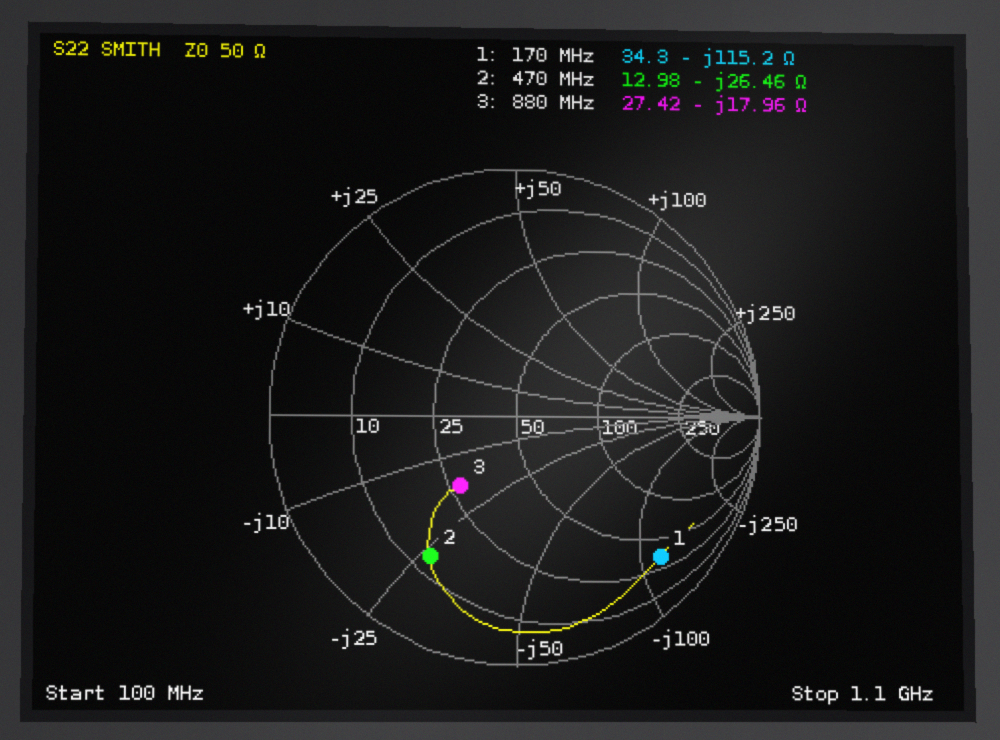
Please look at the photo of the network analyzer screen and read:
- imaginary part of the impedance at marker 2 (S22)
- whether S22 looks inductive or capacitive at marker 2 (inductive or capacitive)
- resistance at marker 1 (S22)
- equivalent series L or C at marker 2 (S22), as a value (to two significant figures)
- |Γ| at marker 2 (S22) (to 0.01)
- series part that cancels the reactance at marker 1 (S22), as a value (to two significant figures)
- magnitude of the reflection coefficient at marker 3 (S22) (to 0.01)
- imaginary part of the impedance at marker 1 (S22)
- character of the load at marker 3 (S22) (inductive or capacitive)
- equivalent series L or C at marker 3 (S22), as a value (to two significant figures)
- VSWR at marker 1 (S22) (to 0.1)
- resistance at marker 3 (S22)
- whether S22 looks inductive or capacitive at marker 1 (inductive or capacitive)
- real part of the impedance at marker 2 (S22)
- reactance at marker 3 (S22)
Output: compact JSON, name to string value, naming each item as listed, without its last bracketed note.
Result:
{"imaginary part of the impedance at marker 2": "-26.46 Ω", "whether S22 looks inductive or capacitive at marker 2": "capacitive", "resistance at marker 1": "34.3 Ω", "equivalent series L or C at marker 2 (S22), as a value": "13 pF", "|Γ| at marker 2 (S22)": "0.67", "series part that cancels the reactance at marker 1 (S22), as a value": "110 nH", "magnitude of the reflection coefficient at marker 3 (S22)": "0.36", "imaginary part of the impedance at marker 1": "-115.2 Ω", "character of the load at marker 3 (S22)": "capacitive", "equivalent series L or C at marker 3 (S22), as a value": "10 pF", "VSWR at marker 1 (S22)": "9.8", "resistance at marker 3": "27.42 Ω", "whether S22 looks inductive or capacitive at marker 1": "capacitive", "real part of the impedance at marker 2": "12.98 Ω", "reactance at marker 3": "-17.96 Ω"}
